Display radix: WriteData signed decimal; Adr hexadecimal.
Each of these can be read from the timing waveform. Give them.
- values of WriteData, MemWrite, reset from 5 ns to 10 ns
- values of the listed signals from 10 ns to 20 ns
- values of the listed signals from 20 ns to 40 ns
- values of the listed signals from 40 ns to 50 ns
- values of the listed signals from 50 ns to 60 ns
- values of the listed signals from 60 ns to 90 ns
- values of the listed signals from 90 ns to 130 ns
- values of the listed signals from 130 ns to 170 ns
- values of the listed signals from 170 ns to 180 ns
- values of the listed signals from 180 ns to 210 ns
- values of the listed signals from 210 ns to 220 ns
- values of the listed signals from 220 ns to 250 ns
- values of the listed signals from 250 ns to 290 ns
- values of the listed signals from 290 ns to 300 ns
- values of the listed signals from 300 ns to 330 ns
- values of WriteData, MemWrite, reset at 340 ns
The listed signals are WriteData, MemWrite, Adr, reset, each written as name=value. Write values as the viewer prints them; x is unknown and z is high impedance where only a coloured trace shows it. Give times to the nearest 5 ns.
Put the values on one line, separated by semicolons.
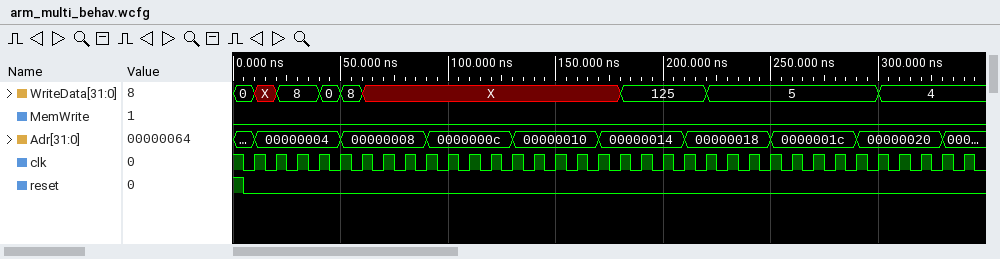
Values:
WriteData=0, MemWrite=0, reset=0; WriteData=X, MemWrite=0, Adr=00000004, reset=0; WriteData=8, MemWrite=0, Adr=00000004, reset=0; WriteData=0, MemWrite=0, Adr=00000004, reset=0; WriteData=8, MemWrite=0, Adr=00000008, reset=0; WriteData=X, MemWrite=0, Adr=00000008, reset=0; WriteData=X, MemWrite=0, Adr=0000000c, reset=0; WriteData=X, MemWrite=0, Adr=00000010, reset=0; WriteData=X, MemWrite=0, Adr=00000014, reset=0; WriteData=125, MemWrite=0, Adr=00000014, reset=0; WriteData=125, MemWrite=0, Adr=00000018, reset=0; WriteData=5, MemWrite=0, Adr=00000018, reset=0; WriteData=5, MemWrite=0, Adr=0000001c, reset=0; WriteData=5, MemWrite=0, Adr=00000020, reset=0; WriteData=4, MemWrite=0, Adr=00000020, reset=0; WriteData=4, MemWrite=0, reset=0
